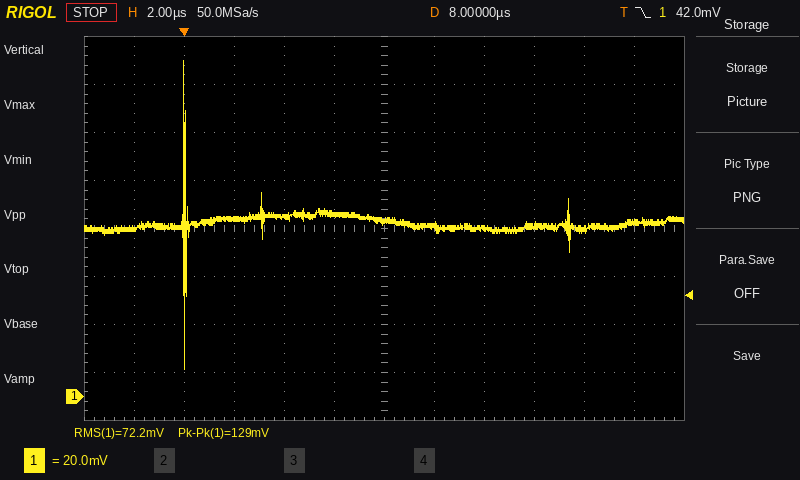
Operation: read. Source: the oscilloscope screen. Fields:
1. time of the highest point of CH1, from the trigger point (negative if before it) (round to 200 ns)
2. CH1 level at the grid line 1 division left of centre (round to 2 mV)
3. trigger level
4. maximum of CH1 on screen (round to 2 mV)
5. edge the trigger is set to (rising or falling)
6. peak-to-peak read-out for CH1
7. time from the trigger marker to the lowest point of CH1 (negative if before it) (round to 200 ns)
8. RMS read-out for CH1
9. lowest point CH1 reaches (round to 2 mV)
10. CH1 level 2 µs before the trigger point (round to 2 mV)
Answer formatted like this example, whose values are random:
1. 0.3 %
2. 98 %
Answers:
1. 0.0 µs
2. 76 mV
3. 42.0 mV
4. 140 mV
5. falling
6. 129 mV
7. 0.0 µs
8. 72.2 mV
9. 12 mV
10. 70 mV
